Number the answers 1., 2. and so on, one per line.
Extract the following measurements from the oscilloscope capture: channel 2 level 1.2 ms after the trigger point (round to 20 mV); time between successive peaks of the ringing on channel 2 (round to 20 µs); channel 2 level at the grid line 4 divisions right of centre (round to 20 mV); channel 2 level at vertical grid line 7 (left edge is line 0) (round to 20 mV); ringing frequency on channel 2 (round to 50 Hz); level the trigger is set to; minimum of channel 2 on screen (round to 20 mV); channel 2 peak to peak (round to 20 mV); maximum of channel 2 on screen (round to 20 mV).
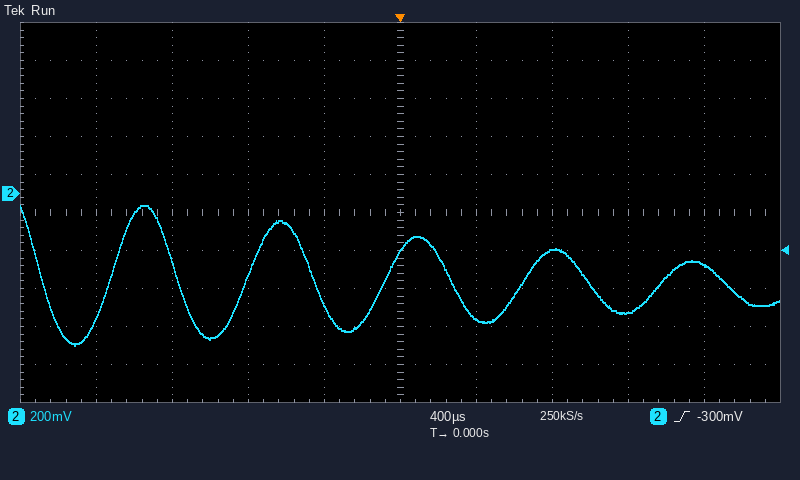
1. -620 mV
2. 720 µs
3. -380 mV
4. -300 mV
5. 1.40 kHz
6. -300 mV
7. -800 mV
8. 740 mV
9. -60 mV
